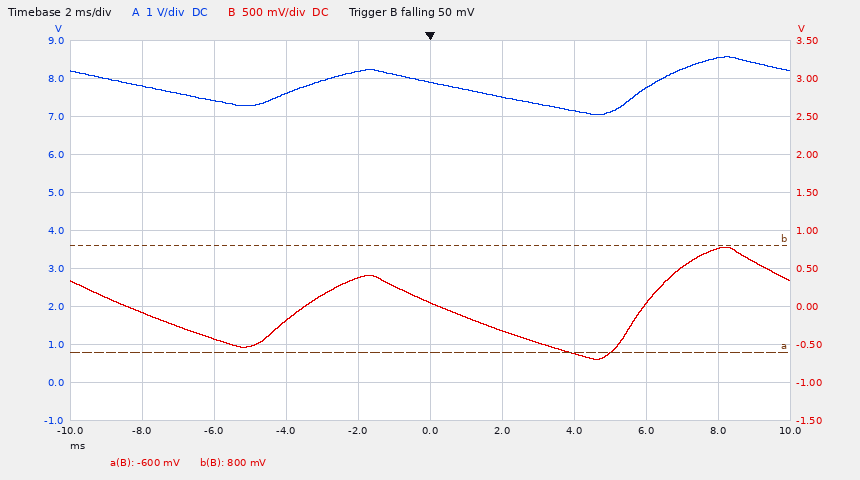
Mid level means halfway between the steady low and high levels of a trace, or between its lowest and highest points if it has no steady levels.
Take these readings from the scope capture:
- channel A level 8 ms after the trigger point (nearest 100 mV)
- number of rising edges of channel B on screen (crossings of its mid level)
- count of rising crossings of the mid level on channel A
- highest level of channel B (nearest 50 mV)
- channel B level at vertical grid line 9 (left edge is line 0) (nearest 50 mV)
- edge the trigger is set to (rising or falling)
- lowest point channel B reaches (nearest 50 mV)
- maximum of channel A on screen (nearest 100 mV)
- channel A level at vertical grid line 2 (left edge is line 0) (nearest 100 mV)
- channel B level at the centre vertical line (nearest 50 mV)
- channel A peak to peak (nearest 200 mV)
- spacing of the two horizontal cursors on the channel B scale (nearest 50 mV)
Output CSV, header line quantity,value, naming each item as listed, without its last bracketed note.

quantity,value
channel A level 8 ms after the trigger point,8.5 V
number of rising edges of channel B on screen,2
count of rising crossings of the mid level on channel A,2
highest level of channel B,800 mV
channel B level at vertical grid line 9 (left edge is line 0),750 mV
edge the trigger is set to,falling
lowest point channel B reaches,-700 mV
maximum of channel A on screen,8.6 V
channel A level at vertical grid line 2 (left edge is line 0),7.4 V
channel B level at the centre vertical line,50 mV
channel A peak to peak,1.6 V
spacing of the two horizontal cursors on the channel B scale,1.40 V
